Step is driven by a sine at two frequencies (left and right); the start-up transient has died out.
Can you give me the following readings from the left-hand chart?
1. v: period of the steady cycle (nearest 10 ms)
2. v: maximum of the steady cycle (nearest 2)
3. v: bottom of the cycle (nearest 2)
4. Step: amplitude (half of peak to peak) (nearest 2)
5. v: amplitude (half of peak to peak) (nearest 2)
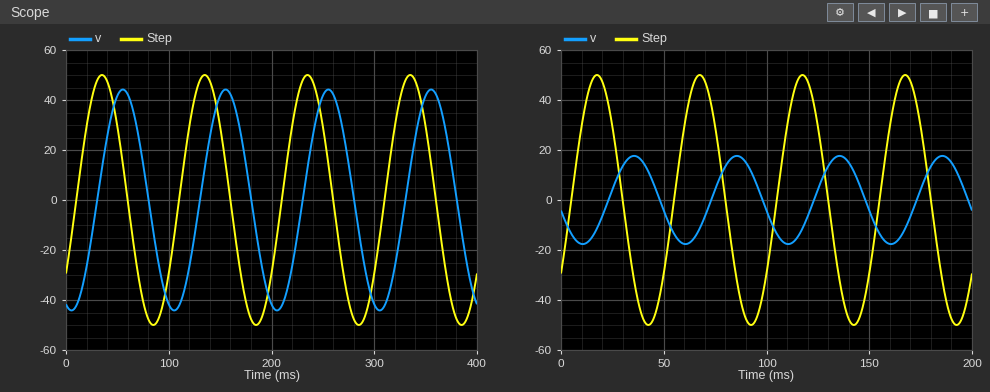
100 ms
44
-44
50
44
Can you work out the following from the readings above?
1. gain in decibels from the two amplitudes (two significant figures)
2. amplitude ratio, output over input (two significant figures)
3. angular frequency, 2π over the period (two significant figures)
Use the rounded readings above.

-1.1 dB
0.88
0.063 rad/ms
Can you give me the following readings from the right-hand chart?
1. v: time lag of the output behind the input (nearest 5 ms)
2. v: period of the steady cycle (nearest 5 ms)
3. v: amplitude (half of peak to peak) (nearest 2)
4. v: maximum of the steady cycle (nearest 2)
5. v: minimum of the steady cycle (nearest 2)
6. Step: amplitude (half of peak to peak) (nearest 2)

20 ms
50 ms
18
18
-18
50
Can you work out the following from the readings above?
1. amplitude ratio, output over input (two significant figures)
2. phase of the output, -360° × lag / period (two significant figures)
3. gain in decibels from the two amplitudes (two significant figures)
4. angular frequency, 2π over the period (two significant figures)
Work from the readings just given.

0.36
-140°
-8.9 dB
0.13 rad/ms
